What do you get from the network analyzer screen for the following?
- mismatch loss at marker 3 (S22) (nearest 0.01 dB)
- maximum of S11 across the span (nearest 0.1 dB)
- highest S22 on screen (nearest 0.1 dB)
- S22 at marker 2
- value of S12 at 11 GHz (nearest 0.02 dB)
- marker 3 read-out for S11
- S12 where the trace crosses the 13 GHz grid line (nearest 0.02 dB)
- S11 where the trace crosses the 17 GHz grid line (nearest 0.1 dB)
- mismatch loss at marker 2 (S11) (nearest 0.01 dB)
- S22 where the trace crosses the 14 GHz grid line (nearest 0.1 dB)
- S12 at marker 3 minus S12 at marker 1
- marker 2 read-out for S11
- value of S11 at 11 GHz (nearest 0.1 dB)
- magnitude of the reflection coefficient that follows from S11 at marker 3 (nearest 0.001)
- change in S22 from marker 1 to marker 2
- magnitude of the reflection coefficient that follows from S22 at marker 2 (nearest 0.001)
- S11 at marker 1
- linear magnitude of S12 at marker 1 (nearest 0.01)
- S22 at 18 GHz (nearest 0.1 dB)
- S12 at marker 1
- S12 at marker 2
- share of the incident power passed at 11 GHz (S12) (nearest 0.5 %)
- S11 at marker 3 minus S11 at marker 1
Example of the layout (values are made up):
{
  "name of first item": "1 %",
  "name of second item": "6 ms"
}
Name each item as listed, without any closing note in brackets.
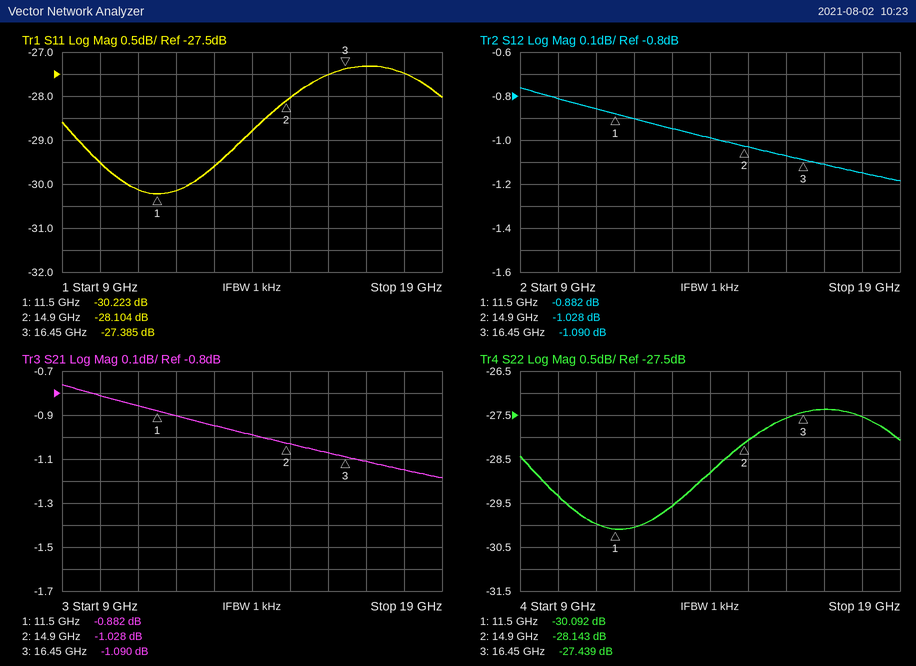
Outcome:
{
  "mismatch loss at marker 3 (S22)": "0.01 dB",
  "maximum of S11 across the span": "-27.3 dB",
  "highest S22 on screen": "-27.4 dB",
  "S22 at marker 2": "-28.143 dB",
  "value of S12 at 11 GHz": "-0.86 dB",
  "marker 3 read-out for S11": "-27.385 dB",
  "S12 where the trace crosses the 13 GHz grid line": "-0.94 dB",
  "S11 where the trace crosses the 17 GHz grid line": "-27.3 dB",
  "mismatch loss at marker 2 (S11)": "0.01 dB",
  "S22 where the trace crosses the 14 GHz grid line": "-28.8 dB",
  "S12 at marker 3 minus S12 at marker 1": "-0.208 dB",
  "marker 2 read-out for S11": "-28.104 dB",
  "value of S11 at 11 GHz": "-30.1 dB",
  "magnitude of the reflection coefficient that follows from S11 at marker 3": "0.043",
  "change in S22 from marker 1 to marker 2": "1.949 dB",
  "magnitude of the reflection coefficient that follows from S22 at marker 2": "0.039",
  "S11 at marker 1": "-30.223 dB",
  "linear magnitude of S12 at marker 1": "0.90",
  "S22 at 18 GHz": "-27.5 dB",
  "S12 at marker 1": "-0.882 dB",
  "S12 at marker 2": "-1.028 dB",
  "share of the incident power passed at 11 GHz (S12)": "82.0 %",
  "S11 at marker 3 minus S11 at marker 1": "2.838 dB"
}
